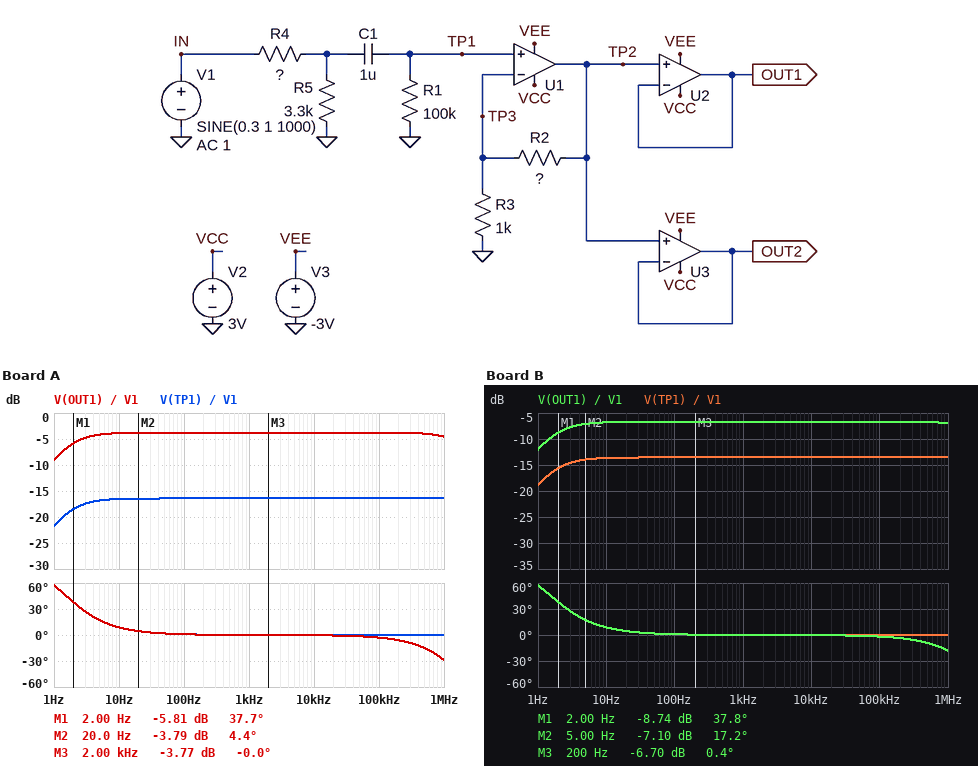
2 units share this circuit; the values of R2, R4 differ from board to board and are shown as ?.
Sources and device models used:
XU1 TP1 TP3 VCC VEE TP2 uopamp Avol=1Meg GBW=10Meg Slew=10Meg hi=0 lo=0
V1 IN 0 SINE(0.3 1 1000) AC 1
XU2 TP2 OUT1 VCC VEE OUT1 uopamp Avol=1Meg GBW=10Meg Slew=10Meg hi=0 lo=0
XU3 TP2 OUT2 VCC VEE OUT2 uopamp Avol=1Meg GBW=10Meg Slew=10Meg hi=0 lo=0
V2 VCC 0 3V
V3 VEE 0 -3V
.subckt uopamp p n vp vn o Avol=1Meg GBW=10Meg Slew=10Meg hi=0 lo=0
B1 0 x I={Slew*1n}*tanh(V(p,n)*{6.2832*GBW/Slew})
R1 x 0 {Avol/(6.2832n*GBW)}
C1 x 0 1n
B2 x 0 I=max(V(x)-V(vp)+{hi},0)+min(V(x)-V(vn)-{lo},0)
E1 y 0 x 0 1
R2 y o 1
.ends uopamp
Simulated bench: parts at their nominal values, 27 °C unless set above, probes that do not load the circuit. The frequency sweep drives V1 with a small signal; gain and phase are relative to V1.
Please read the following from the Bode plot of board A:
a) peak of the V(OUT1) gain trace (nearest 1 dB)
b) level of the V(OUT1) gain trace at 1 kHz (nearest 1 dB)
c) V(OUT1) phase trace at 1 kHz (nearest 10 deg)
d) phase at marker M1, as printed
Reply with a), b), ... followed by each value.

a) -4 dB
b) -4 dB
c) 0 deg
d) 37.7 deg
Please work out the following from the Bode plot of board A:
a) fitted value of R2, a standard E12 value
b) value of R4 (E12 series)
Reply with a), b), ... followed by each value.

a) 3.3 kΩ
b) 18 kΩ
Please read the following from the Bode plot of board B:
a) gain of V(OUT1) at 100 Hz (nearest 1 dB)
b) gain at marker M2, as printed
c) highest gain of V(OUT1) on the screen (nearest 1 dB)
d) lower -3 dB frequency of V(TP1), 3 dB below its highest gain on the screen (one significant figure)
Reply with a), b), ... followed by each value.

a) -7 dB
b) -7.10 dB
c) -7 dB
d) 2 Hz
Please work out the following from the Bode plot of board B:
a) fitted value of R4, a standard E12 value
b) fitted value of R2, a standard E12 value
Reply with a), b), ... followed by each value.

a) 12 kΩ
b) 1.2 kΩ
